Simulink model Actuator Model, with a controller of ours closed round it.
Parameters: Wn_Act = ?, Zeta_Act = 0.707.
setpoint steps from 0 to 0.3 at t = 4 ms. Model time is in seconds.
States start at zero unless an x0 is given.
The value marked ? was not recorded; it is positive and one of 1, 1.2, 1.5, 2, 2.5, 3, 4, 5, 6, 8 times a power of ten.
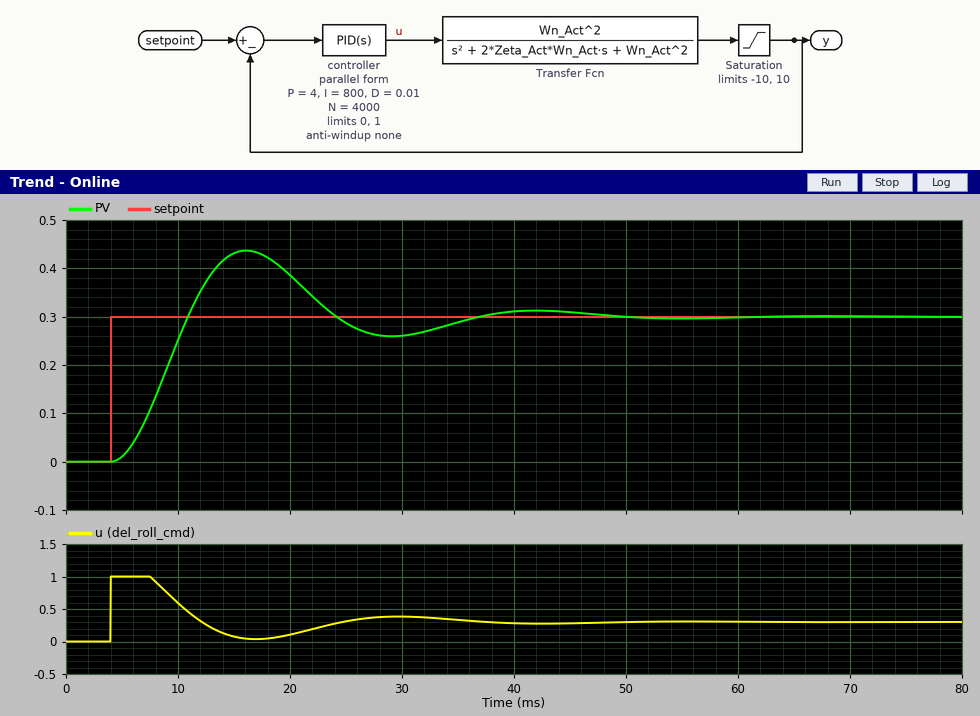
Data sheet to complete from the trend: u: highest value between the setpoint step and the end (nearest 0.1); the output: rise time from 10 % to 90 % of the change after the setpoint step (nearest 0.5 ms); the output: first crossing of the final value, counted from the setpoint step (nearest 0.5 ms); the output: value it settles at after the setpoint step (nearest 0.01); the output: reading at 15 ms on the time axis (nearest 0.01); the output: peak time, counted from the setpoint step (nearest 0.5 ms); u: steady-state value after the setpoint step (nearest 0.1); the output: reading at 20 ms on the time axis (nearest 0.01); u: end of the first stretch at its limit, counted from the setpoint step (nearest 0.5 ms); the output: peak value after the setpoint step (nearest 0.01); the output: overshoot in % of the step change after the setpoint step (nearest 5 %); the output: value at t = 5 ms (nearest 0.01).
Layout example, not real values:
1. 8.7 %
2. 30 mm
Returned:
1. 1.0
2. 4.5 ms
3. 7.0 ms
4. 0.30
5. 0.43
6. 12.0 ms
7. 0.3
8. 0.39
9. 3.5 ms
10. 0.44
11. 45 %
12. 0.01
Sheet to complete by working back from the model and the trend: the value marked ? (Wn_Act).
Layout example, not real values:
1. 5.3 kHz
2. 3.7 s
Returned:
1. 150
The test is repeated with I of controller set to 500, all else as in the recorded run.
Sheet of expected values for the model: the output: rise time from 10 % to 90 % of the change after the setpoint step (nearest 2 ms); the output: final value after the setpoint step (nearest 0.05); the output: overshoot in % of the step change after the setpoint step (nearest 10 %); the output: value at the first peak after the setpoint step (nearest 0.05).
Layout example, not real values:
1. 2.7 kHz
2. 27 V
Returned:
1. 6 ms
2. 0.30
3. 30 %
4. 0.40
